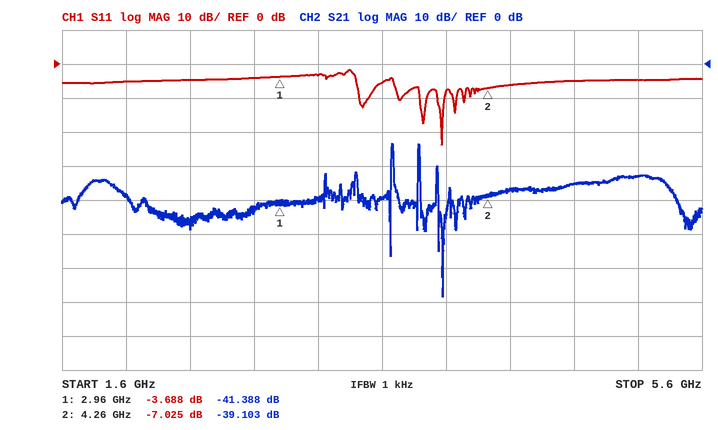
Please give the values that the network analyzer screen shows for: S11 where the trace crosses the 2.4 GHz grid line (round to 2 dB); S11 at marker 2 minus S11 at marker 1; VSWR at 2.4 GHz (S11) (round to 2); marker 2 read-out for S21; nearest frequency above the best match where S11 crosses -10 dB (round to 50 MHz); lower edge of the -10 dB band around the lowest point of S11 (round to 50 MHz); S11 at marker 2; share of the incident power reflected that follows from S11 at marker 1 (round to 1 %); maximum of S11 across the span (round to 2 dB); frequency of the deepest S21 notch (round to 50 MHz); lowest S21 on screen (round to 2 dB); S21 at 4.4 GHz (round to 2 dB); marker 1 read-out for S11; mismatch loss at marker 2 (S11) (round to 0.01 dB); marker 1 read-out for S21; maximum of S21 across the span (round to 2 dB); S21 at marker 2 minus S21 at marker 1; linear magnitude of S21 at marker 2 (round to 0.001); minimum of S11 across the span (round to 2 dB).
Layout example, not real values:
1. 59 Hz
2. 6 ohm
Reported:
1. -4 dB
2. -3.337 dB
3. 4
4. -39.103 dB
5. 4.00 GHz
6. 3.95 GHz
7. -7.025 dB
8. 43 %
9. -2 dB
10. 4.00 GHz
11. -68 dB
12. -36 dB
13. -3.688 dB
14. 0.96 dB
15. -41.388 dB
16. -24 dB
17. 2.285 dB
18. 0.011
19. -24 dB
